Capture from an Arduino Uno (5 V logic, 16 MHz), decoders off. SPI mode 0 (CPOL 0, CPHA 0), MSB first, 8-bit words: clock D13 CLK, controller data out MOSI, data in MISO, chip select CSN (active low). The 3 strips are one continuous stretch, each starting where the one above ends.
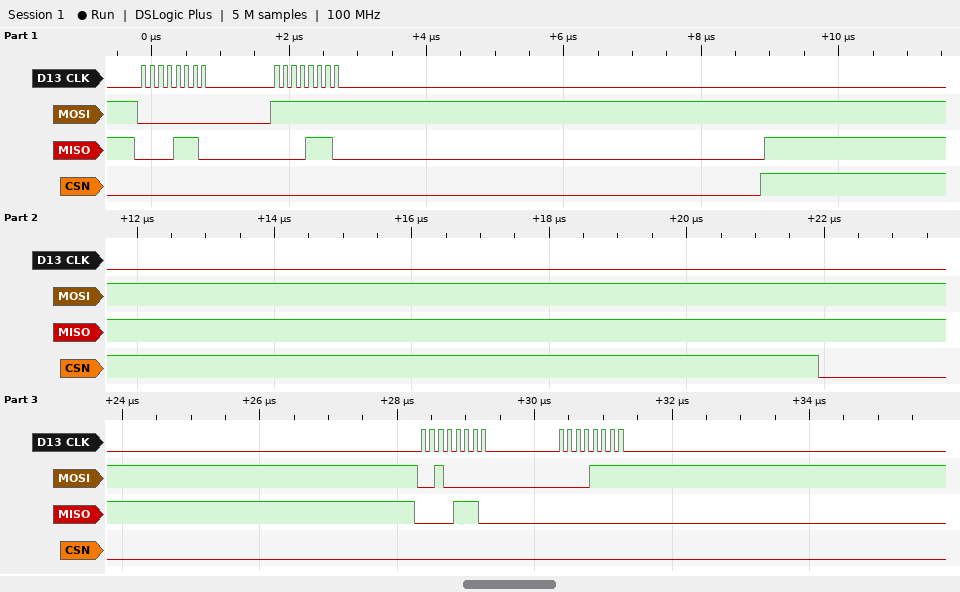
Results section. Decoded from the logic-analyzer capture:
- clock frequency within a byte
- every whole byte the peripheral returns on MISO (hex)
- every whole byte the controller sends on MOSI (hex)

8 MHz
0E 0E 0E 00
00 FF 20 0F
